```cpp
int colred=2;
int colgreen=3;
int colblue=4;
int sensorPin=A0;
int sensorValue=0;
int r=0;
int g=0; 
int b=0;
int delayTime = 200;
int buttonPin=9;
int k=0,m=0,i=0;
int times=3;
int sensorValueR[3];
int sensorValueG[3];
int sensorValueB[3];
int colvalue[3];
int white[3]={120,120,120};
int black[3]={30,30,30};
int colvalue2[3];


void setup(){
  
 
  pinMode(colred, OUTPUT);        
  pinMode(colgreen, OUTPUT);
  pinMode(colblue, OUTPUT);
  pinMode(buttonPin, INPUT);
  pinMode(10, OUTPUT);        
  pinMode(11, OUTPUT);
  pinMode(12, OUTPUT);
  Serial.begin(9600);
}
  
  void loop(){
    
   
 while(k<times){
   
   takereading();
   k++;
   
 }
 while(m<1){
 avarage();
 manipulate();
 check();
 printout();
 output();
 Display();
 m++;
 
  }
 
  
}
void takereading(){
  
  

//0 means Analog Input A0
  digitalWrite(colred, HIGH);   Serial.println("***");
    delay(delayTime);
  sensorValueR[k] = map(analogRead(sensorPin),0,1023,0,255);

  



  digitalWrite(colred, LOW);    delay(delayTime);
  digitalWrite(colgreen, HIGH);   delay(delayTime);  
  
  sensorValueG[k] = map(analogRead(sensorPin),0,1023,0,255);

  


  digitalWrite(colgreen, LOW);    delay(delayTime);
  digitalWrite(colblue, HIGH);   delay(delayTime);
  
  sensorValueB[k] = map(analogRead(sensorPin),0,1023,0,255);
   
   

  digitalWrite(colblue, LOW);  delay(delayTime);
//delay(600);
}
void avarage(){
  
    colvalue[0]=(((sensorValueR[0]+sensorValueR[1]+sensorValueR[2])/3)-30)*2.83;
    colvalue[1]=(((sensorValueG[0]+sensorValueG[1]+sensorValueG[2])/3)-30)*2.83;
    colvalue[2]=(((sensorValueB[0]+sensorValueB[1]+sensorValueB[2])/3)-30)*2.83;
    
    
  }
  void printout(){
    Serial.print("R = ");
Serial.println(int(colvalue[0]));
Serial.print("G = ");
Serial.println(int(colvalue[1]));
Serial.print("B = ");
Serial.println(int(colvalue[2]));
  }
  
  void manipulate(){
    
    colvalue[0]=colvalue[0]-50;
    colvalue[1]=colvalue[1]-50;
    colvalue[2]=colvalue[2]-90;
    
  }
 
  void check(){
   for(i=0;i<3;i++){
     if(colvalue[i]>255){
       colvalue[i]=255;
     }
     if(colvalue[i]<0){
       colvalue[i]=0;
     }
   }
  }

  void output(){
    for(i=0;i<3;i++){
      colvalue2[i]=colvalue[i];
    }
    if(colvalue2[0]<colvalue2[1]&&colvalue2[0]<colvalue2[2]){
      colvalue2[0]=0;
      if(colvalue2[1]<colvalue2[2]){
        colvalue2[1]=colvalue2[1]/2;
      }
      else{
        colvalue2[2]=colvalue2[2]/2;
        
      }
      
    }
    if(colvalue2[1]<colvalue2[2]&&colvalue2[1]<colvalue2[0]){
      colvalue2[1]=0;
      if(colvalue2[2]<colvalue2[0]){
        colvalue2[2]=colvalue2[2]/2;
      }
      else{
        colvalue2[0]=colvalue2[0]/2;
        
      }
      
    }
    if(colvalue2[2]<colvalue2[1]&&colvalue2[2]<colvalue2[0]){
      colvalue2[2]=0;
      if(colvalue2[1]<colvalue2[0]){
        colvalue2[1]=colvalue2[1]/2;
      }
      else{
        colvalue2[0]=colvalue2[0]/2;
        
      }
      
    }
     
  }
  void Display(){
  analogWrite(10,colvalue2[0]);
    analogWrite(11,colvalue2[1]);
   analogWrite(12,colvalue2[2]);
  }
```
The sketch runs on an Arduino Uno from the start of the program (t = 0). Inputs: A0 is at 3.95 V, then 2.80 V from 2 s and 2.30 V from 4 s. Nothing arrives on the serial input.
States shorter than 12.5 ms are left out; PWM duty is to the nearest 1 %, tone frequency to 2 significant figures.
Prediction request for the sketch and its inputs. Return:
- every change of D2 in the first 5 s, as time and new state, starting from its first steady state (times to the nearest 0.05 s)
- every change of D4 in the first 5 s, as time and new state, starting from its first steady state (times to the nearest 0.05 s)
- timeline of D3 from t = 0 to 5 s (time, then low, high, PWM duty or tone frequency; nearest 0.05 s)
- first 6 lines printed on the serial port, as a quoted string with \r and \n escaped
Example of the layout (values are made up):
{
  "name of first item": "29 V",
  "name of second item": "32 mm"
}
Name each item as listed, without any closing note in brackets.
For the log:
{
  "every change of D2 in the first 5 s, as time and new state, starting from its first steady state": "0 s high; 0.2 s low; 1.2 s high; 1.4 s low; 2.4 s high; 2.6 s low",
  "every change of D4 in the first 5 s, as time and new state, starting from its first steady state": "0 s low; 0.8 s high; 1 s low; 2 s high; 2.2 s low; 3.2 s high; 3.4 s low",
  "timeline of D3 from t = 0 to 5 s": "0 s low; 0.4 s high; 0.6 s low; 1.6 s high; 1.8 s low; 2.8 s high; 3 s low",
  "first 6 lines printed on the serial port, as a quoted string with \\r and \\n escaped": "\"***\\r\\n***\\r\\n***\\r\\nR = 255\\r\\nG = 255\\r\\nB = 255\\r\\n\""
}
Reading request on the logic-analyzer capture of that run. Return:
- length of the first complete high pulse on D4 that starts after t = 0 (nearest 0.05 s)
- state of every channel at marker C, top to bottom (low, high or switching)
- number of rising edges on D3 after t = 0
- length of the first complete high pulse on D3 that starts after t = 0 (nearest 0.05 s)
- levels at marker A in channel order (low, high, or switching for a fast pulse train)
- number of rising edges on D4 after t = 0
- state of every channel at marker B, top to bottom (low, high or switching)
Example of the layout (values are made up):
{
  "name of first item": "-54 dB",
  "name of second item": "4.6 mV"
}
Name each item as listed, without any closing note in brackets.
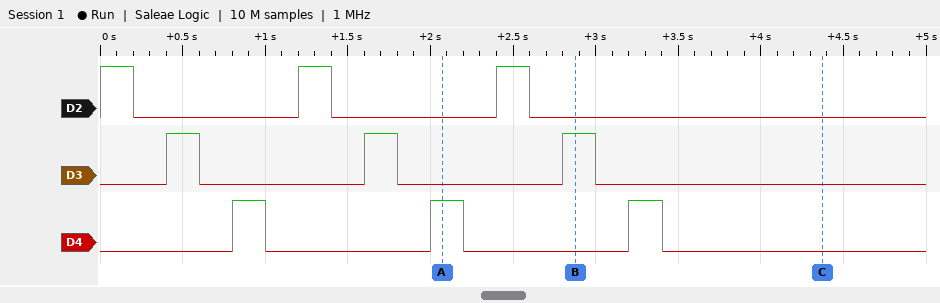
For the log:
{
  "length of the first complete high pulse on D4 that starts after t = 0": "0.20 s",
  "state of every channel at marker C, top to bottom": "D2 low, D3 low, D4 low",
  "number of rising edges on D3 after t = 0": "3",
  "length of the first complete high pulse on D3 that starts after t = 0": "0.20 s",
  "levels at marker A in channel order": "D2 low, D3 low, D4 high",
  "number of rising edges on D4 after t = 0": "3",
  "state of every channel at marker B, top to bottom": "D2 low, D3 high, D4 low"
}
